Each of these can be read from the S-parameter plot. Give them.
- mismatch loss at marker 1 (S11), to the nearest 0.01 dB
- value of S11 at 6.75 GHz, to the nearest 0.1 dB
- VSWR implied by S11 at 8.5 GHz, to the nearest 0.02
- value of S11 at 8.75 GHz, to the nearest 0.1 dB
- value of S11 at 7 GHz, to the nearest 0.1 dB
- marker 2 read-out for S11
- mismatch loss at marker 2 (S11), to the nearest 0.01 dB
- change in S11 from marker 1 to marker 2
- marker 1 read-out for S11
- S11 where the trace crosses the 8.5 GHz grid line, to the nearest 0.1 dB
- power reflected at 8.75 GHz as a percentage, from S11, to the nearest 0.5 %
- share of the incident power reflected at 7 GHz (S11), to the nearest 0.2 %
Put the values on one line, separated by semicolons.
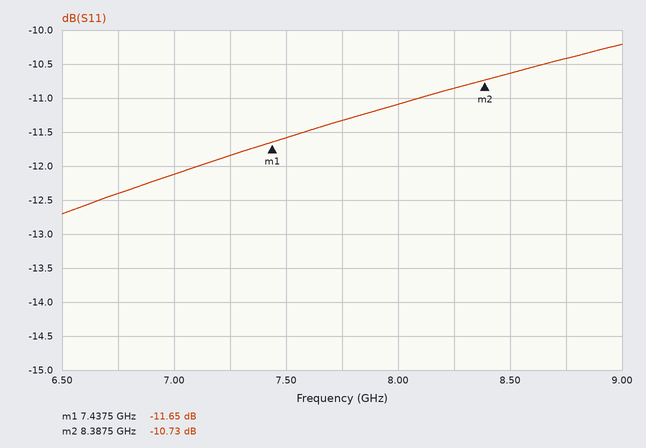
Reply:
0.31 dB; -12.4 dB; 1.84; -10.4 dB; -12.1 dB; -10.73 dB; 0.38 dB; 0.92 dB; -11.65 dB; -10.6 dB; 9.0 %; 6.2 %
